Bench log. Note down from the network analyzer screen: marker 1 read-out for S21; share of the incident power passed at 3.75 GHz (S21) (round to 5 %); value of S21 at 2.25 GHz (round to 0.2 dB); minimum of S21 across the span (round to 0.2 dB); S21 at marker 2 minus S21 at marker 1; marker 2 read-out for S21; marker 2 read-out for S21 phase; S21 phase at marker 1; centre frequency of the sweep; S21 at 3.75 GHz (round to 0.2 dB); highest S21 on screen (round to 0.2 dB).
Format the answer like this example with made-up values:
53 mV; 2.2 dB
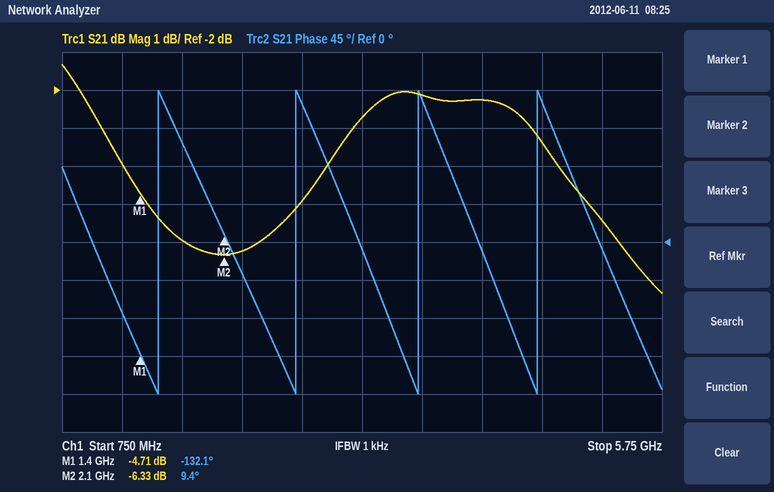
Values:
-4.71 dB; 60 %; -6.2 dB; -7.4 dB; -1.62 dB; -6.33 dB; 9.4°; -132.1°; 3.25 GHz; -2.2 dB; -1.4 dB
